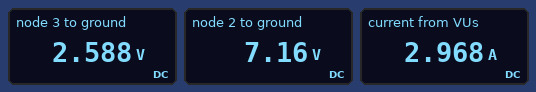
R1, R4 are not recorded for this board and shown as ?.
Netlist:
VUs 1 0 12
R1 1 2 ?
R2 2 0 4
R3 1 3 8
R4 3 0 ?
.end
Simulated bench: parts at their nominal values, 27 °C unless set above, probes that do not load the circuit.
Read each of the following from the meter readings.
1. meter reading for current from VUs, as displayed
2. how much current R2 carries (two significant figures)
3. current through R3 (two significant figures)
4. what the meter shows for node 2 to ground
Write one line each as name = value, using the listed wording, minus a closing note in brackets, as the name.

meter reading for current from VUs, as displayed = 2.968 A
how much current R2 carries = 1.8 A
current through R3 = 1.2 A
what the meter shows for node 2 to ground = 7.16 V
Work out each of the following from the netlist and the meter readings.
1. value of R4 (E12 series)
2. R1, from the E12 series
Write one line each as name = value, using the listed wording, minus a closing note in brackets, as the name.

value of R4 = 2.2 Ω
R1, from the E12 series = 2.7 Ω
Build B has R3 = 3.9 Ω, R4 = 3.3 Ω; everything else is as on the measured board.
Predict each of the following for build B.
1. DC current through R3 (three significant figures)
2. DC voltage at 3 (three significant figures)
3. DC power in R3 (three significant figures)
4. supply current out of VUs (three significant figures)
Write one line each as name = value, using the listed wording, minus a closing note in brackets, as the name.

DC current through R3 = 1.67 A
DC voltage at 3 = 5.50 V
DC power in R3 = 10.8 W
supply current out of VUs = 3.46 A
